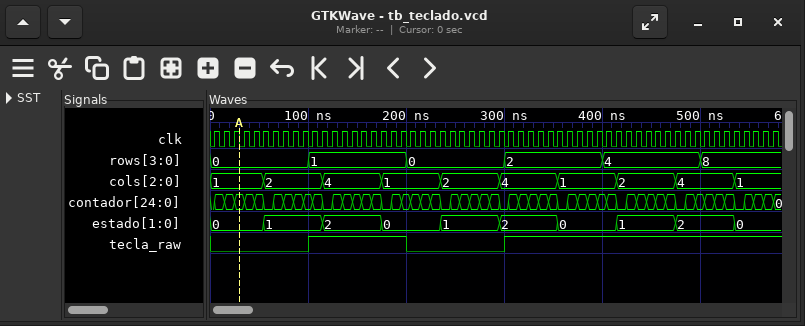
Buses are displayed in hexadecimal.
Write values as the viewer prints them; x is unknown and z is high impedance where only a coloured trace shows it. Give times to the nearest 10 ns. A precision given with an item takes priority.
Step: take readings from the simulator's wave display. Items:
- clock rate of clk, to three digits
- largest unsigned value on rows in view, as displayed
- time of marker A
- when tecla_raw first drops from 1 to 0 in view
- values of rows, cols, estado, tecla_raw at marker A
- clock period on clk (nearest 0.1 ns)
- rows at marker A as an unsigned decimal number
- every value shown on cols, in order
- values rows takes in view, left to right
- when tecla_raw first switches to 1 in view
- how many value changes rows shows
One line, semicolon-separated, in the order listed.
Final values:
100 MHz; 8; 30 ns; 200 ns; rows=0, cols=1, estado=0, tecla_raw=0; 10 ns; 0; 1, 2, 4, 1, 2, 4, 1, 2, 4, 1; 0, 1, 0, 2, 4, 8; 100 ns; 5
